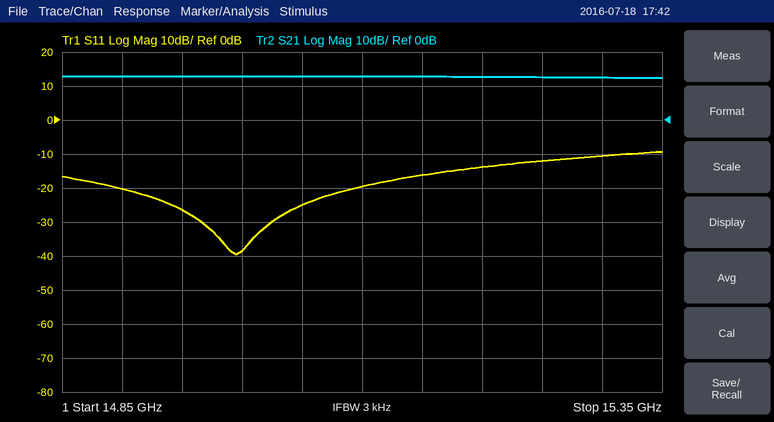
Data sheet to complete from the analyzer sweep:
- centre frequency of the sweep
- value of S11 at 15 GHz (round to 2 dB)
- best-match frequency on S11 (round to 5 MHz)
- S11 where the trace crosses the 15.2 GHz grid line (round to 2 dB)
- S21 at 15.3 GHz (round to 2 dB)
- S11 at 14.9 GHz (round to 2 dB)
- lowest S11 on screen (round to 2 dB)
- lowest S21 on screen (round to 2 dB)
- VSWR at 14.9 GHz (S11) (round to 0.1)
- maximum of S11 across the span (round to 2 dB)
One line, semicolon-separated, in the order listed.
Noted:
15.1 GHz; -38 dB; 14.995 GHz; -14 dB; 12 dB; -20 dB; -40 dB; 12 dB; 1.2; -10 dB
